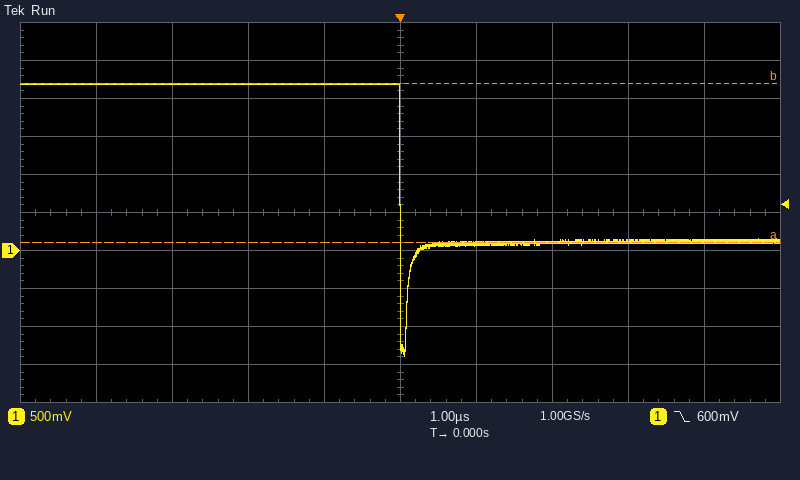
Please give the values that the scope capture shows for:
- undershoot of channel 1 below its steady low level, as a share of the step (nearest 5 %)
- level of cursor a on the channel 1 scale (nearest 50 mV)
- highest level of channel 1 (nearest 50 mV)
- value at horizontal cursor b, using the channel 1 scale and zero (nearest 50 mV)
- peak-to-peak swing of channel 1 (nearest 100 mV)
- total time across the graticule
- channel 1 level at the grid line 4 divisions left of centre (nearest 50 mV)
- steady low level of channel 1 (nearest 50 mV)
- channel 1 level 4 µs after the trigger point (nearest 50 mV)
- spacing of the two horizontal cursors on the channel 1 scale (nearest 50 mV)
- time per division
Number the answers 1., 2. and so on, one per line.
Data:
1. 70 %
2. 100 mV
3. 2.20 V
4. 2.20 V
5. 3.60 V
6. 10 µs
7. 2.20 V
8. 100 mV
9. 100 mV
10. 2.10 V
11. 1 µs
